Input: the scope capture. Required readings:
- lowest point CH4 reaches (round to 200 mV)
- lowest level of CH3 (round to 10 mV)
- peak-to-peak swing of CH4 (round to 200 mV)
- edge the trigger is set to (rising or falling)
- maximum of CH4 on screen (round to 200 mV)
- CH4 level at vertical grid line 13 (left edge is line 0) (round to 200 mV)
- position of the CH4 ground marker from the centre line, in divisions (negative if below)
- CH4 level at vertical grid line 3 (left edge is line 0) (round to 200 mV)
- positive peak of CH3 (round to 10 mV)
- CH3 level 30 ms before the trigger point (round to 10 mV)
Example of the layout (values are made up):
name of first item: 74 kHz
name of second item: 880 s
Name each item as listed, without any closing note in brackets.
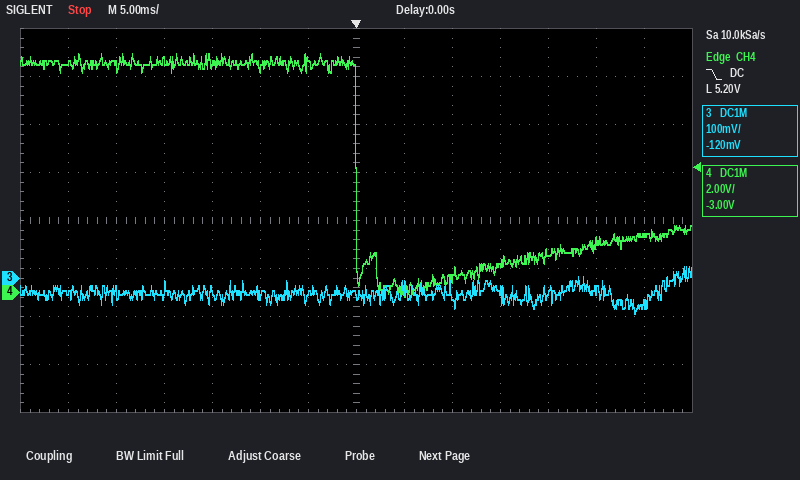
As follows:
lowest point CH4 reaches: -200 mV
lowest level of CH3: -70 mV
peak-to-peak swing of CH4: 10.2 V
edge the trigger is set to: falling
maximum of CH4 on screen: 10.0 V
CH4 level at vertical grid line 13 (left edge is line 0): 2.4 V
position of the CH4 ground marker from the centre line, in divisions: -1.5 div
CH4 level at vertical grid line 3 (left edge is line 0): 9.6 V
positive peak of CH3: 20 mV
CH3 level 30 ms before the trigger point: -30 mV
